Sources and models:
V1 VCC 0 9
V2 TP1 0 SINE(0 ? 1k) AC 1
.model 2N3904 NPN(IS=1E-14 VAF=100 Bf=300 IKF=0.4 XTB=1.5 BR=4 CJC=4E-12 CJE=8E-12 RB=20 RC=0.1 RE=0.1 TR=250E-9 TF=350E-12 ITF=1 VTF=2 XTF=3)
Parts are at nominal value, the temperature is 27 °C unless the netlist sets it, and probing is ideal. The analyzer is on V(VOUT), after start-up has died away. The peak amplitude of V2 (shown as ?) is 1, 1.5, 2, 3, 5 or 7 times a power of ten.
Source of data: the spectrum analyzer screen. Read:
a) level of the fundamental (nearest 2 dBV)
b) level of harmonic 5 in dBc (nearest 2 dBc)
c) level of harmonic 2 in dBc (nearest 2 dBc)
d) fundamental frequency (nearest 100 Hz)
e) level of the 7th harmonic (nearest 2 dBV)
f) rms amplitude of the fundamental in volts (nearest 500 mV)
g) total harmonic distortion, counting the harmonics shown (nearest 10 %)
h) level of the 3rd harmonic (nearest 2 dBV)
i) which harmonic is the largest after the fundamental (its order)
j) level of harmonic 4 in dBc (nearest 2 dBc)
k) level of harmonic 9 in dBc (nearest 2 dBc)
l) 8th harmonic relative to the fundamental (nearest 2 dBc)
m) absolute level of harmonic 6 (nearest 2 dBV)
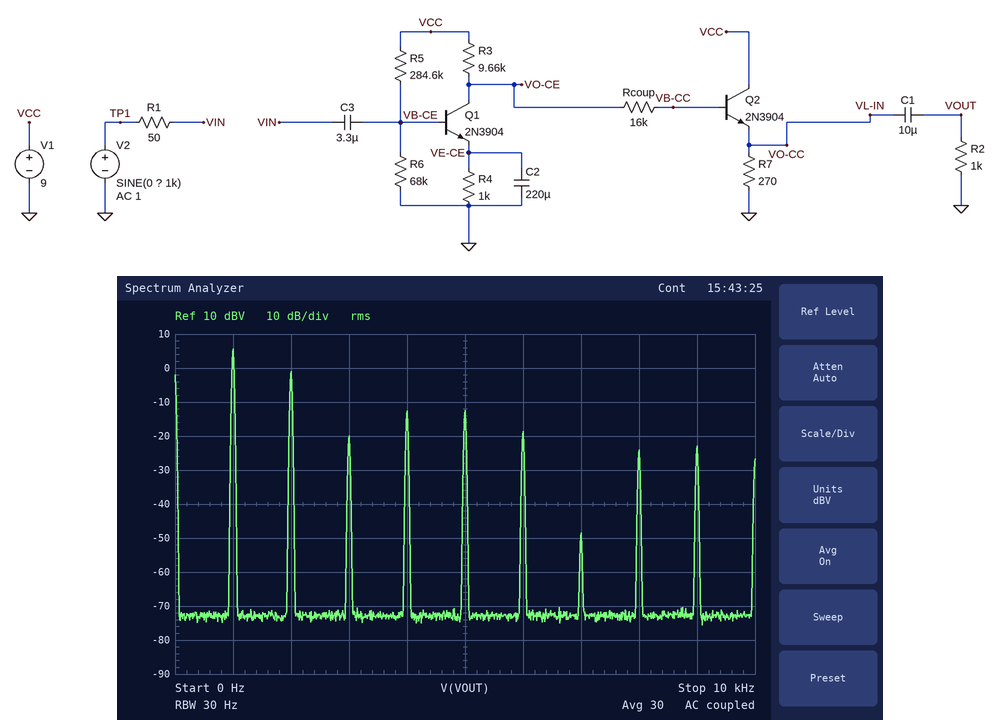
6 dBV
-18 dBc
-6 dBc
1.0 kHz
-48 dBV
2.0 V
50 %
-20 dBV
2
-18 dBc
-28 dBc
-30 dBc
-18 dBV
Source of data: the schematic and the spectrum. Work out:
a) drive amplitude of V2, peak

100 mV
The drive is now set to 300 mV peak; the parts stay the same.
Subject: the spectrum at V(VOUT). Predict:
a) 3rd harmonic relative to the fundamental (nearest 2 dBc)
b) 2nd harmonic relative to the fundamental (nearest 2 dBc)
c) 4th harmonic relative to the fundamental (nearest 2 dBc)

-6 dBc
-2 dBc
-14 dBc
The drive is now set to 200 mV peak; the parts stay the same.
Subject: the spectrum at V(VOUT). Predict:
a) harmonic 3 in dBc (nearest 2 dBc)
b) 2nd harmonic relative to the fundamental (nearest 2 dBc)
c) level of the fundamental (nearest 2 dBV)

-10 dBc
-4 dBc
4 dBV
